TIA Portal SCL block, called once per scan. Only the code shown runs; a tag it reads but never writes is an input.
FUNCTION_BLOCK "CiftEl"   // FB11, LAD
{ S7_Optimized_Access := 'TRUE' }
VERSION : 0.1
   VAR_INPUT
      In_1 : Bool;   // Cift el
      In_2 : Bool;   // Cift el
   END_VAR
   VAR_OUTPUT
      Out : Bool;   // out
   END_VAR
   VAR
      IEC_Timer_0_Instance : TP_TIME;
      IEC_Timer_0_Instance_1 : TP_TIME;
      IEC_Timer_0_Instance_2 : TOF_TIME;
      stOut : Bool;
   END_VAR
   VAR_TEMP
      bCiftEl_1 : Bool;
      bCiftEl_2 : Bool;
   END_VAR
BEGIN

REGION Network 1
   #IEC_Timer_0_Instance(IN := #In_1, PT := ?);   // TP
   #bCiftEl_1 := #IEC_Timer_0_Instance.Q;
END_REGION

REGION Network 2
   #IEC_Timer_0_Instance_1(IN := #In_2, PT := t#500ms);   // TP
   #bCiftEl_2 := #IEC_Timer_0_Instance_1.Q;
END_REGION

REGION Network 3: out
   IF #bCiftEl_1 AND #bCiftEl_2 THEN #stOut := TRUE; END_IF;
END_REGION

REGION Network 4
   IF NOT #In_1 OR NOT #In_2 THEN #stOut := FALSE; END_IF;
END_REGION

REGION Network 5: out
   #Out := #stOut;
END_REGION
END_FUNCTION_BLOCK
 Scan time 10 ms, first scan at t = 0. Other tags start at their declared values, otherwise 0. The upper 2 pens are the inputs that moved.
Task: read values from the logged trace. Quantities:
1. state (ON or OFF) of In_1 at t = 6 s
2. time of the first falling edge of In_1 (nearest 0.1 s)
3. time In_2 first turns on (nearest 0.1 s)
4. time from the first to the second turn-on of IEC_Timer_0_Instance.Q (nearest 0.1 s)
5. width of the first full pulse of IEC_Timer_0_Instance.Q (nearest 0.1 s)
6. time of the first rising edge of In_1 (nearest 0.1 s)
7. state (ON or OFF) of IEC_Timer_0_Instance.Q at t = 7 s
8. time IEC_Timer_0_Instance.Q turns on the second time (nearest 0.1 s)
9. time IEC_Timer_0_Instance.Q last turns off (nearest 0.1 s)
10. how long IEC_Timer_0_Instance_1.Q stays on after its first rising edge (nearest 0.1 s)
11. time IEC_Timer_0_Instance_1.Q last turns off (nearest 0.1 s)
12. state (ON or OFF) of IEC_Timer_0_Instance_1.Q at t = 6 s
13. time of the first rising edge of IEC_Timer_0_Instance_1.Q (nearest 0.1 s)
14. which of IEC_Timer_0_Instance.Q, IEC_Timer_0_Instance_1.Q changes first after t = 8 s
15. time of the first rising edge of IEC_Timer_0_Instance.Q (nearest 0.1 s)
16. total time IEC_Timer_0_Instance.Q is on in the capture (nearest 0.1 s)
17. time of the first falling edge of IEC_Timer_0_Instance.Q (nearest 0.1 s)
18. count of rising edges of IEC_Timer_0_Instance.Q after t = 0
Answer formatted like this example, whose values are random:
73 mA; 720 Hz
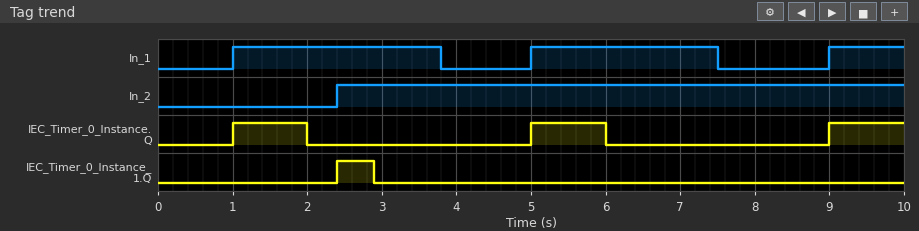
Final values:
ON; 3.8 s; 2.4 s; 4.0 s; 1.0 s; 1.0 s; OFF; 5.0 s; 6.0 s; 0.5 s; 2.9 s; OFF; 2.4 s; IEC_Timer_0_Instance.Q; 1.0 s; 3.0 s; 2.0 s; 3
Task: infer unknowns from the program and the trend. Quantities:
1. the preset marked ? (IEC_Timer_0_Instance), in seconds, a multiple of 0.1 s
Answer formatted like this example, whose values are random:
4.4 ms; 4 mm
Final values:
1.0 s
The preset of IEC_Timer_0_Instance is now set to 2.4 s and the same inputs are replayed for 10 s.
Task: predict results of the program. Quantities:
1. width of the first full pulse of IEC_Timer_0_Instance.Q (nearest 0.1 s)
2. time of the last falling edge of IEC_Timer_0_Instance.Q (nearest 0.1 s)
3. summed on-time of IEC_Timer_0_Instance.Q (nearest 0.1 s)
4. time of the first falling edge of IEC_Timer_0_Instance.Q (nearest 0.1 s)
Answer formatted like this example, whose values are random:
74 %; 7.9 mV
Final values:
2.4 s; 7.4 s; 5.8 s; 3.4 s
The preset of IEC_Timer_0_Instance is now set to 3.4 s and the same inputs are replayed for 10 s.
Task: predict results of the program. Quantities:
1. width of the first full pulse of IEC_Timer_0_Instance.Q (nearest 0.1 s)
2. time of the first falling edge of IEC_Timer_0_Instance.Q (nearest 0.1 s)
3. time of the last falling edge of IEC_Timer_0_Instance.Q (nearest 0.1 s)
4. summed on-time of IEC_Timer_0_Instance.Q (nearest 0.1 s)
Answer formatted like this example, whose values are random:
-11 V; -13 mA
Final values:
3.4 s; 4.4 s; 8.4 s; 7.8 s
